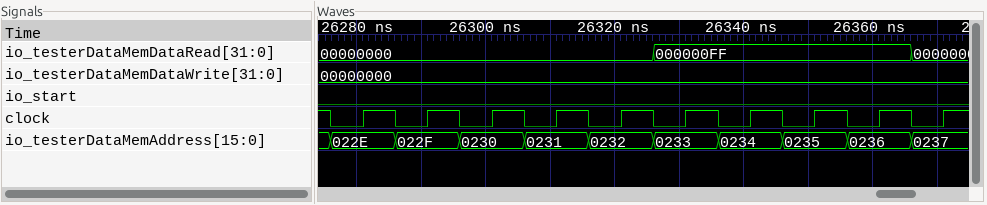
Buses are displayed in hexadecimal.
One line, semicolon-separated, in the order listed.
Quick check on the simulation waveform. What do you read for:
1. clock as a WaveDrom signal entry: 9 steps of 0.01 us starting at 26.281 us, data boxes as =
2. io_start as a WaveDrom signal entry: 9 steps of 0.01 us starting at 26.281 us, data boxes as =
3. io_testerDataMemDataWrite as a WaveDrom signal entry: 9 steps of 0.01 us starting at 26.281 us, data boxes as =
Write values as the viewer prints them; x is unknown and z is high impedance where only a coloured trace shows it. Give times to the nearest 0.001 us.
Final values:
{name: 'clock', wave: 'p........'}; {name: 'io_start', wave: '0........'}; {name: 'io_testerDataMemDataWrite', wave: '=........', data: '00000000'}
